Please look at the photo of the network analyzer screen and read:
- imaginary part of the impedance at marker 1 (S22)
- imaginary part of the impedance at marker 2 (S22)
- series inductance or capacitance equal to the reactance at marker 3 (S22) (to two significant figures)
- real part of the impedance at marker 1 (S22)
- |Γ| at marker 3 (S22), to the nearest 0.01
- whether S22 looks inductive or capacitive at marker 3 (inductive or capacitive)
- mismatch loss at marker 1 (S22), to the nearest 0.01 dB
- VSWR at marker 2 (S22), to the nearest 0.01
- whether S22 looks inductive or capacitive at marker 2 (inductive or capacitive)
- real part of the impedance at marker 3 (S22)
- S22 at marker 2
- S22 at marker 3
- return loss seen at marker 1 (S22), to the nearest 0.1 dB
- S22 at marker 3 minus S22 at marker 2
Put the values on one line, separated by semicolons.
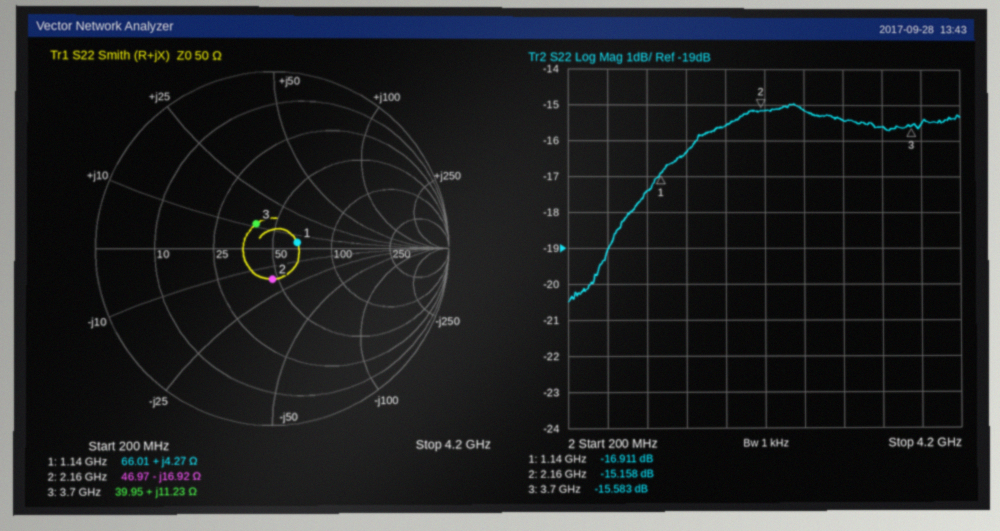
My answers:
+4.27 Ω; -16.92 Ω; 480 pH; 66.01 Ω; 0.17; inductive; 0.09 dB; 1.42; capacitive; 39.95 Ω; -15.158 dB; -15.583 dB; 16.9 dB; -0.425 dB
